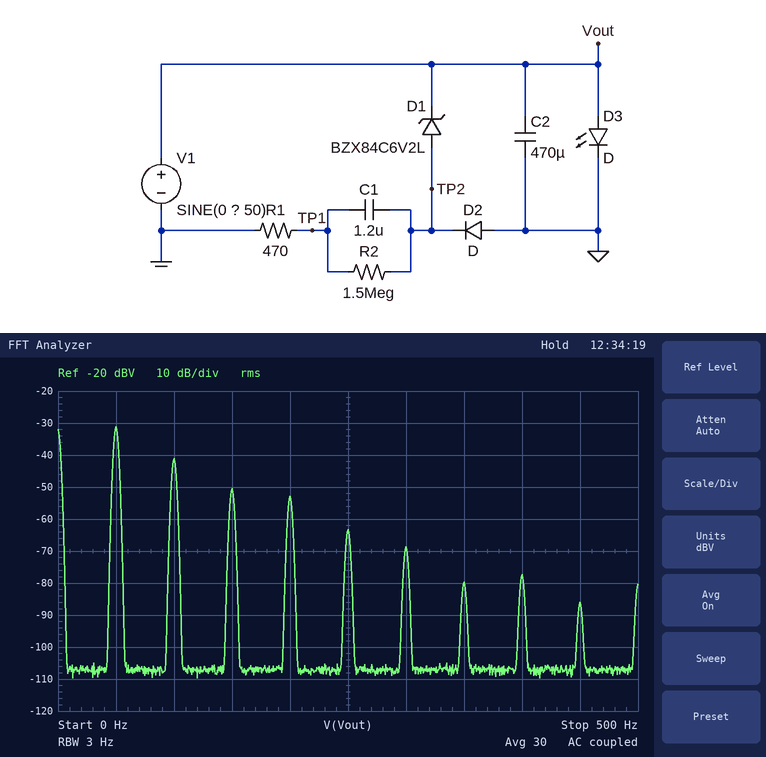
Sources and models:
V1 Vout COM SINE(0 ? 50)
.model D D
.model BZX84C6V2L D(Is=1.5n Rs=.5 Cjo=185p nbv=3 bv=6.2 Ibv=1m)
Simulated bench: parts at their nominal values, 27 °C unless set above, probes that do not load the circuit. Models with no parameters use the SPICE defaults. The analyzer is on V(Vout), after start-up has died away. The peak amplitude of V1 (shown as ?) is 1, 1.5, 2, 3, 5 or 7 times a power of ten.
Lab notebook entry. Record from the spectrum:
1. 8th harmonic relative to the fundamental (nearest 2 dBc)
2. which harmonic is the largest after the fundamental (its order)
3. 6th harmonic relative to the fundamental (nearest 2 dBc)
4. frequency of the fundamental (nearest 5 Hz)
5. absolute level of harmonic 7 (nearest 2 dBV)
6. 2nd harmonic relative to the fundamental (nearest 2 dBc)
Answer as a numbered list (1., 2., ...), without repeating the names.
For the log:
1. -46 dBc
2. 2
3. -38 dBc
4. 50 Hz
5. -80 dBV
6. -10 dBc
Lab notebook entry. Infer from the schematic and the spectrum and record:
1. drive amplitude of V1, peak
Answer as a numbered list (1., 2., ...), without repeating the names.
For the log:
1. 70 V
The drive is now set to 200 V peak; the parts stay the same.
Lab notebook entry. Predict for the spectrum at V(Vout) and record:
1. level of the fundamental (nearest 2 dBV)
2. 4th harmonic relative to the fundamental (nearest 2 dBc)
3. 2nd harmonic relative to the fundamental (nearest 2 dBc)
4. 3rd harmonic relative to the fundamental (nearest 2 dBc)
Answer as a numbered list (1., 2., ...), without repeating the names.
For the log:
1. -28 dBV
2. -18 dBc
3. -12 dBc
4. -16 dBc
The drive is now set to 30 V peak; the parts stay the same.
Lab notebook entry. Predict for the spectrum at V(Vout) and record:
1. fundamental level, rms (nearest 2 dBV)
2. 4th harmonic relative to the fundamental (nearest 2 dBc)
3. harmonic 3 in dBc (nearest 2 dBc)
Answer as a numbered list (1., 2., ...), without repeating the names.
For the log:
1. -34 dBV
2. -30 dBc
3. -24 dBc
